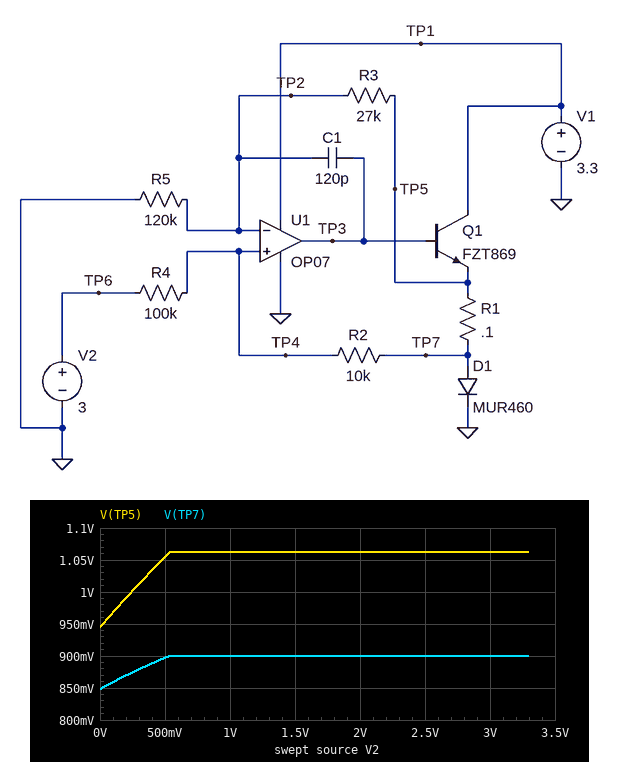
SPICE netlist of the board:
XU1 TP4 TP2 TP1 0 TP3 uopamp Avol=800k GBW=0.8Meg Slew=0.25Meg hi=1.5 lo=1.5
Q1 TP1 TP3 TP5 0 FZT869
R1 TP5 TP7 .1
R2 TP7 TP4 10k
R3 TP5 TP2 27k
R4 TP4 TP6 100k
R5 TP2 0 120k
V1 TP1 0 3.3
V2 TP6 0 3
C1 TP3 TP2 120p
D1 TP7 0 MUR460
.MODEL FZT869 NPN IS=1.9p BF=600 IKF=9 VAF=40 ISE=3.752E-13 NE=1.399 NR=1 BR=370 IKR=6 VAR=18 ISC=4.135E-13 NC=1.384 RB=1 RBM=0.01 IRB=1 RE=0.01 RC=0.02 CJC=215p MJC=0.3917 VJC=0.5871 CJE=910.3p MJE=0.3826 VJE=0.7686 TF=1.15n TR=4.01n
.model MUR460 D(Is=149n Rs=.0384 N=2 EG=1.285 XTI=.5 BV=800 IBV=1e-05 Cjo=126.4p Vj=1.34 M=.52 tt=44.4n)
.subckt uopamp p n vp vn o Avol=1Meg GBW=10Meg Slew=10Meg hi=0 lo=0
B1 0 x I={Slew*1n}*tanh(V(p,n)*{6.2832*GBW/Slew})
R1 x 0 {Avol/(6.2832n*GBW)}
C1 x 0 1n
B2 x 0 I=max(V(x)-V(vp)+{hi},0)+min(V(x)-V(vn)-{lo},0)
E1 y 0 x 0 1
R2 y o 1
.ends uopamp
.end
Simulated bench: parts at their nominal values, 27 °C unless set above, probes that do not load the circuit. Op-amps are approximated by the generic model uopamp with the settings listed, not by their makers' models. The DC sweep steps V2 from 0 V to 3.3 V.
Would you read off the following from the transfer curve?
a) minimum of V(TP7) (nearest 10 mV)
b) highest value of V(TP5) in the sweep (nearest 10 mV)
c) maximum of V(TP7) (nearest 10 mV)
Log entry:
850 mV
1.06 V
900 mV
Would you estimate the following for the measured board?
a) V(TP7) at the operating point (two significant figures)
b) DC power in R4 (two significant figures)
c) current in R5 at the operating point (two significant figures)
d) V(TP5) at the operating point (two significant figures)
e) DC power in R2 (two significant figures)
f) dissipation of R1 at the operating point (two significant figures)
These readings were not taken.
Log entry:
900 mV
36 µW
7.2 µA
1.1 V
3.6 µW
260 mW
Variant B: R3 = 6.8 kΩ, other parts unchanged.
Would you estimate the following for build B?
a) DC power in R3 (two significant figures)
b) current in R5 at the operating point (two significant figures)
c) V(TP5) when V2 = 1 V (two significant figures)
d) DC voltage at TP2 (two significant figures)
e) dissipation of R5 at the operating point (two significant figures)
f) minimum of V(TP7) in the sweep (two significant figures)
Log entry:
480 nW
8.4 µA
880 mV
1.0 V
8.4 µW
780 mV
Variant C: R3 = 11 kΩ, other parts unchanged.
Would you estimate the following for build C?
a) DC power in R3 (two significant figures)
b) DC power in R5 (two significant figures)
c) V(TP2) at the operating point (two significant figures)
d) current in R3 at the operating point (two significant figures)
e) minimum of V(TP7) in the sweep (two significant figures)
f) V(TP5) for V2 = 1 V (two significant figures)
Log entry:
720 nW
7.9 µW
970 mV
8.1 µA
780 mV
940 mV
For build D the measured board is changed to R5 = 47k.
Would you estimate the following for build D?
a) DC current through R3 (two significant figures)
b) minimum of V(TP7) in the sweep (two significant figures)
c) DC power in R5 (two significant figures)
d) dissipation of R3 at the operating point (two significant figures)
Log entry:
14 µA
900 mV
9.7 µW
5.6 µW
